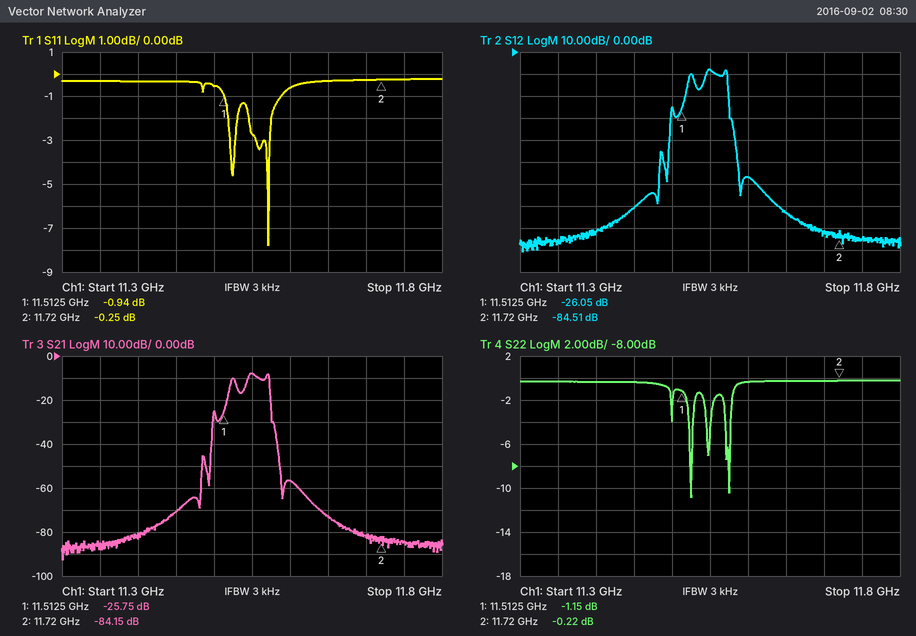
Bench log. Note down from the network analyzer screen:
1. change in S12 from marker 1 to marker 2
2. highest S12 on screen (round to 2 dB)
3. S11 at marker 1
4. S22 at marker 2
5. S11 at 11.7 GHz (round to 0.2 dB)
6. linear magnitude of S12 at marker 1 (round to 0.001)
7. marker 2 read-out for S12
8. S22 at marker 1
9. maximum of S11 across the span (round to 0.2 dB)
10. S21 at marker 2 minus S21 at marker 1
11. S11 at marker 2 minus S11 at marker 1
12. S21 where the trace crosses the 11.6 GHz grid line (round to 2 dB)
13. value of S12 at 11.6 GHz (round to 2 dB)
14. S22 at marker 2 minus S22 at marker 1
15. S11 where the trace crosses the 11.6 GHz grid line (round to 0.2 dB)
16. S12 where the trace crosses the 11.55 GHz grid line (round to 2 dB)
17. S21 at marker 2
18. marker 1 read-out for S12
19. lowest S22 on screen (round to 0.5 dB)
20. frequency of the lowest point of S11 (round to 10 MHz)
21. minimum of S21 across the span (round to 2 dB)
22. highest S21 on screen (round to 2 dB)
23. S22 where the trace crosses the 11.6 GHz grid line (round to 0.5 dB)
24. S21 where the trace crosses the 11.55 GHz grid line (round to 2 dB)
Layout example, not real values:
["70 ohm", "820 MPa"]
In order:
["-58.46 dB", "-8 dB", "-0.94 dB", "-0.22 dB", "-0.2 dB", "0.050", "-84.51 dB", "-1.15 dB", "-0.2 dB", "-58.40 dB", "0.69 dB", "-56 dB", "-56 dB", "0.93 dB", "-0.6 dB", "-8 dB", "-84.15 dB", "-26.05 dB", "-11.0 dB", "11.57 GHz", "-92 dB", "-8 dB", "-0.5 dB", "-8 dB"]
